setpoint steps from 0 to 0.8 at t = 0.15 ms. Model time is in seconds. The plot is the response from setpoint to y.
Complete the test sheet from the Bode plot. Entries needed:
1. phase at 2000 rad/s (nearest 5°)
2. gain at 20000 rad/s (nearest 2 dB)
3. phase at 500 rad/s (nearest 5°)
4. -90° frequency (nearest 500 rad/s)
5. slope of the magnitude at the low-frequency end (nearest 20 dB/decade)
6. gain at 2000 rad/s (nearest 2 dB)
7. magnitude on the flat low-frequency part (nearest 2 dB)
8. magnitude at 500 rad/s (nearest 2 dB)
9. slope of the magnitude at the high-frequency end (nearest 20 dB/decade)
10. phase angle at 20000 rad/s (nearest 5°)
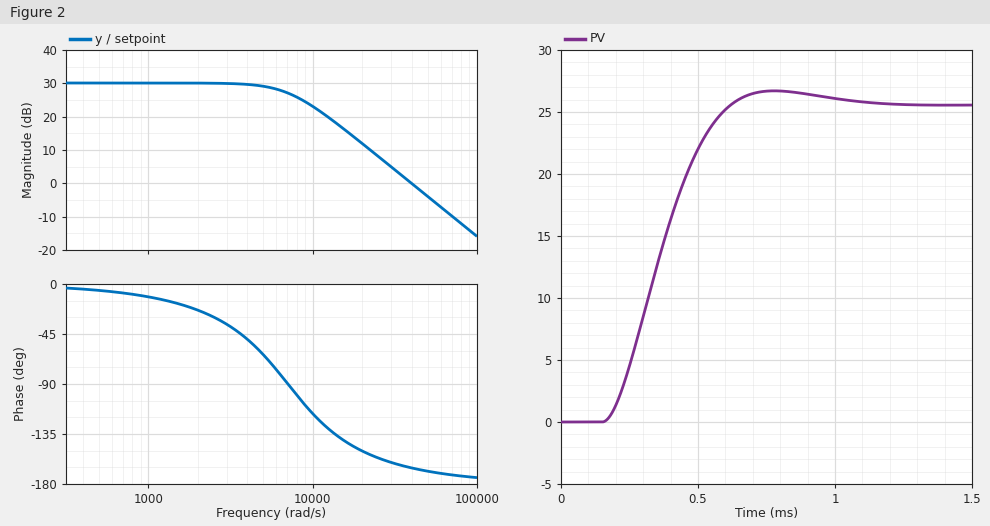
-25°
12 dB
-5°
7000 rad/s
0 dB/decade
30 dB
30 dB
30 dB
-40 dB/decade
-150°
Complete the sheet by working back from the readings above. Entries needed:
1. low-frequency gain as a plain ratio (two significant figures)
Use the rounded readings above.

32
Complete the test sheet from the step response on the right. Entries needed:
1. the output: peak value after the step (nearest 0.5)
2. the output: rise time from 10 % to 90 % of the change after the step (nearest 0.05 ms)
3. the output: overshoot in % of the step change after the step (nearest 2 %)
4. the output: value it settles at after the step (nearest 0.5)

26.5
0.30 ms
4 %
25.5
